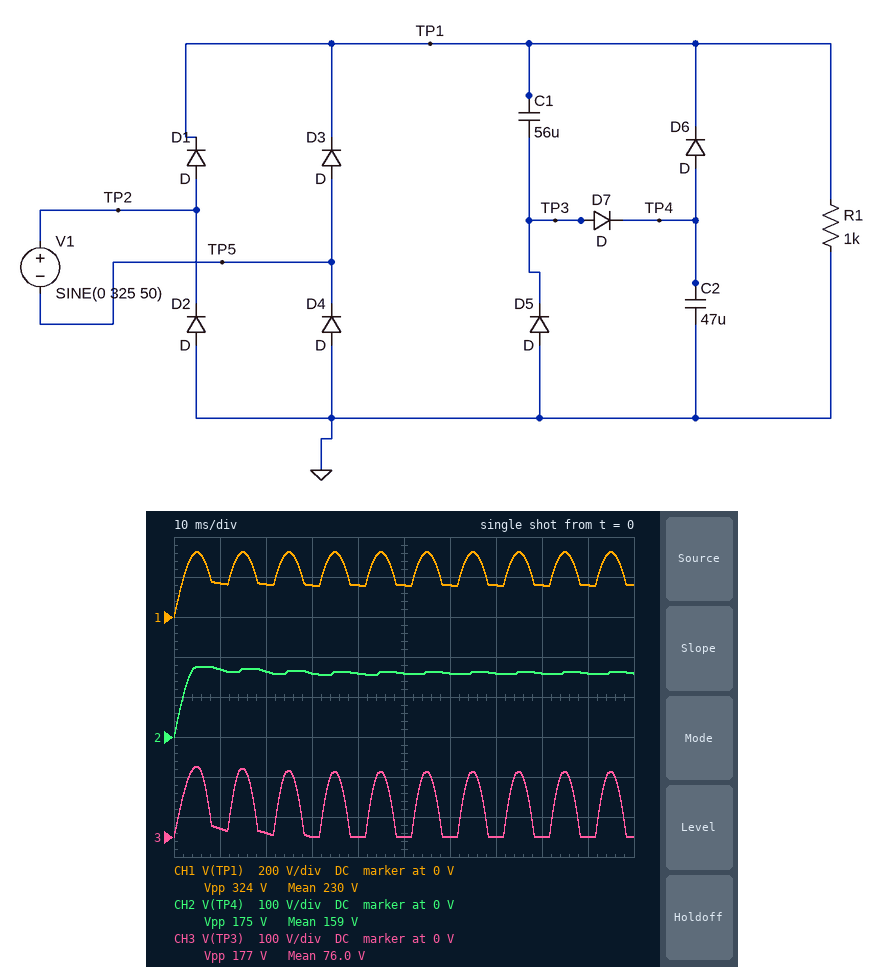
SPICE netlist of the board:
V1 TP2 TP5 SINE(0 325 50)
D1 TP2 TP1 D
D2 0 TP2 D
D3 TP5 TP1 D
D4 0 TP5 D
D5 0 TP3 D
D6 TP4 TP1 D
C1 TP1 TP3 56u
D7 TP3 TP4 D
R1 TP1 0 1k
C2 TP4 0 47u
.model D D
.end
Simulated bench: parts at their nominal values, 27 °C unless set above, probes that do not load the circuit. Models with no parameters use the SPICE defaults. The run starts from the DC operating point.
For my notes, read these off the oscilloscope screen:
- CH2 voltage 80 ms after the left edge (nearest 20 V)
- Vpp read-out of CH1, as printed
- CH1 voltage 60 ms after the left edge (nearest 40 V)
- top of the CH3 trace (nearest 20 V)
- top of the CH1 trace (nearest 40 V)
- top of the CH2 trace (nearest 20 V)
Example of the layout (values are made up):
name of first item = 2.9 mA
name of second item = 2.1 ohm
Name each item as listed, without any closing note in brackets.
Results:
CH2 voltage 80 ms after the left edge = 160 V
Vpp read-out of CH1, as printed = 324 V
CH1 voltage 60 ms after the left edge = 160 V
top of the CH3 trace = 180 V
top of the CH1 trace = 320 V
top of the CH2 trace = 180 V
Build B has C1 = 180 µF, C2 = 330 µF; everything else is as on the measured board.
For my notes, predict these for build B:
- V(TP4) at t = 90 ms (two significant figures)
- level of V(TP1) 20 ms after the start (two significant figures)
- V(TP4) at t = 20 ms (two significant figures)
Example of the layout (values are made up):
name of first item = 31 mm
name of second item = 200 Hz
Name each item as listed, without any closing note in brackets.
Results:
V(TP4) at t = 90 ms = 130 V
level of V(TP1) 20 ms after the start = 200 V
V(TP4) at t = 20 ms = 120 V
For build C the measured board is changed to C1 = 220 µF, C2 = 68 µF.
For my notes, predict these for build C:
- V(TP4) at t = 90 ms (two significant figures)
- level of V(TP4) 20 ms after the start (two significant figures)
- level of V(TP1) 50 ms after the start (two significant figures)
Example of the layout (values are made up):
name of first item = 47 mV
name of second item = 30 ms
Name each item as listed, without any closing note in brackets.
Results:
V(TP4) at t = 90 ms = 210 V
level of V(TP4) 20 ms after the start = 230 V
level of V(TP1) 50 ms after the start = 220 V
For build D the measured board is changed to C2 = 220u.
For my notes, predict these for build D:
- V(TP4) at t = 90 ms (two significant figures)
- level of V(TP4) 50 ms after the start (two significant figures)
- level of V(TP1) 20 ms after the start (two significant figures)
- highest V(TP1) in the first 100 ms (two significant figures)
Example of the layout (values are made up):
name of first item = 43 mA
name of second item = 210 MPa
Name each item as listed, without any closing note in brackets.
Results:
V(TP4) at t = 90 ms = 99 V
level of V(TP4) 50 ms after the start = 84 V
level of V(TP1) 20 ms after the start = 240 V
highest V(TP1) in the first 100 ms = 320 V
